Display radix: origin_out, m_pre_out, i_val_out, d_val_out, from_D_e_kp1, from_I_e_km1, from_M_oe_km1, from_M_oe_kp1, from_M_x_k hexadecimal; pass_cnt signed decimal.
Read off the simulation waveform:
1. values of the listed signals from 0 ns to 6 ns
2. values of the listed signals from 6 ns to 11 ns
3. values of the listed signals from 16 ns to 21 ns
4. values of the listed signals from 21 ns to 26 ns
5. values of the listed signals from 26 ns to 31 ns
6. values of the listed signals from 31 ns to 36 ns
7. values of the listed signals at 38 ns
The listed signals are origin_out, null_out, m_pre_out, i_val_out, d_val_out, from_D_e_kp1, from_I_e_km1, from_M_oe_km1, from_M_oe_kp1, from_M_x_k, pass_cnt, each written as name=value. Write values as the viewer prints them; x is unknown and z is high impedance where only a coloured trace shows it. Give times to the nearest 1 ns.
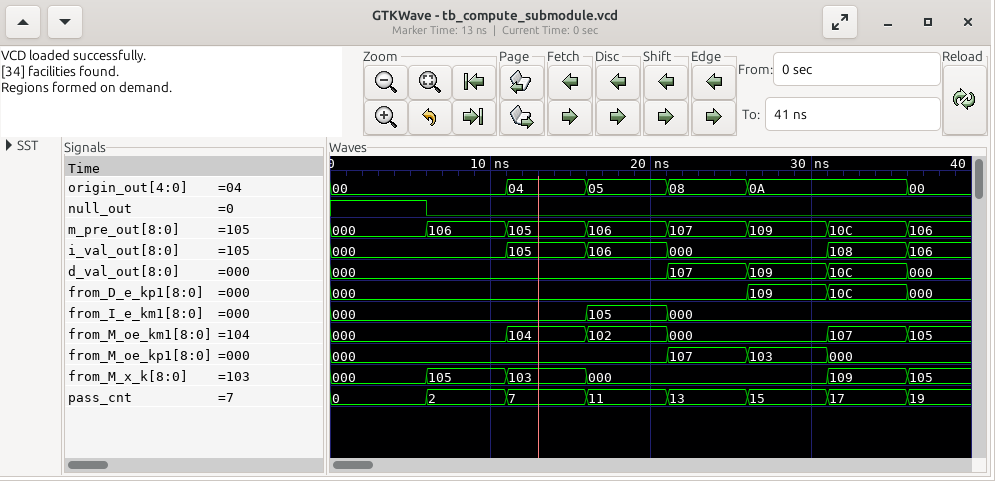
origin_out=00, null_out=1, m_pre_out=000, i_val_out=000, d_val_out=000, from_D_e_kp1=000, from_I_e_km1=000, from_M_oe_km1=000, from_M_oe_kp1=000, from_M_x_k=000, pass_cnt=0
origin_out=00, null_out=0, m_pre_out=106, i_val_out=000, d_val_out=000, from_D_e_kp1=000, from_I_e_km1=000, from_M_oe_km1=000, from_M_oe_kp1=000, from_M_x_k=105, pass_cnt=2
origin_out=05, null_out=0, m_pre_out=106, i_val_out=106, d_val_out=000, from_D_e_kp1=000, from_I_e_km1=105, from_M_oe_km1=102, from_M_oe_kp1=000, from_M_x_k=000, pass_cnt=11
origin_out=08, null_out=0, m_pre_out=107, i_val_out=000, d_val_out=107, from_D_e_kp1=000, from_I_e_km1=000, from_M_oe_km1=000, from_M_oe_kp1=107, from_M_x_k=000, pass_cnt=13
origin_out=0A, null_out=0, m_pre_out=109, i_val_out=000, d_val_out=109, from_D_e_kp1=109, from_I_e_km1=000, from_M_oe_km1=000, from_M_oe_kp1=103, from_M_x_k=000, pass_cnt=15
origin_out=0A, null_out=0, m_pre_out=10C, i_val_out=108, d_val_out=10C, from_D_e_kp1=10C, from_I_e_km1=000, from_M_oe_km1=107, from_M_oe_kp1=000, from_M_x_k=109, pass_cnt=17
origin_out=00, null_out=0, m_pre_out=106, i_val_out=106, d_val_out=000, from_D_e_kp1=000, from_I_e_km1=000, from_M_oe_km1=105, from_M_oe_kp1=000, from_M_x_k=105, pass_cnt=19
